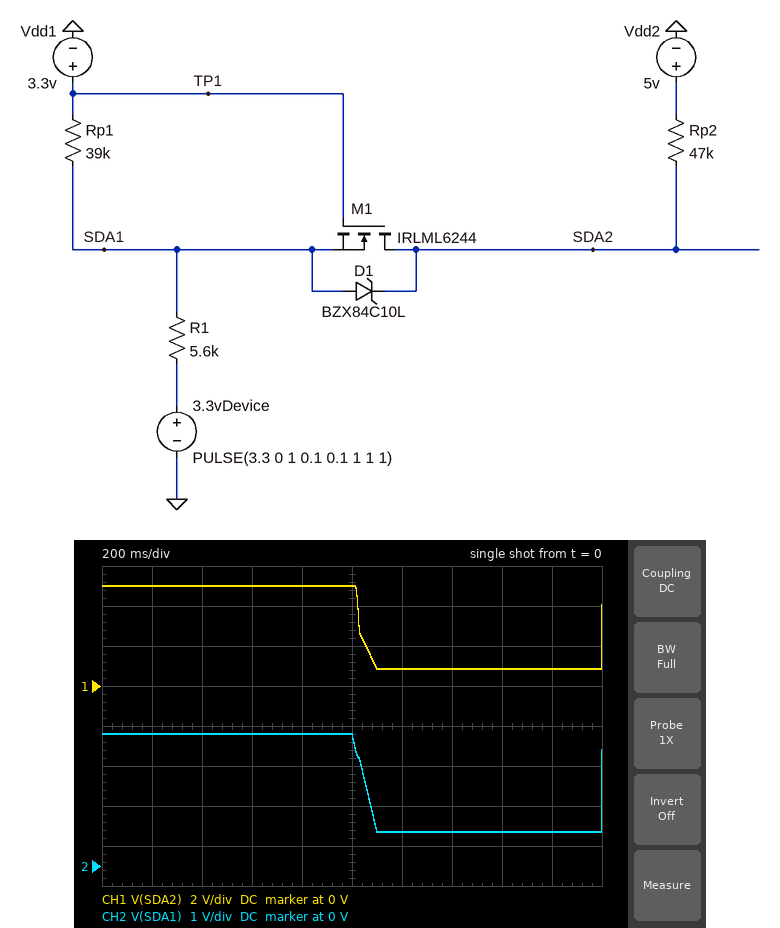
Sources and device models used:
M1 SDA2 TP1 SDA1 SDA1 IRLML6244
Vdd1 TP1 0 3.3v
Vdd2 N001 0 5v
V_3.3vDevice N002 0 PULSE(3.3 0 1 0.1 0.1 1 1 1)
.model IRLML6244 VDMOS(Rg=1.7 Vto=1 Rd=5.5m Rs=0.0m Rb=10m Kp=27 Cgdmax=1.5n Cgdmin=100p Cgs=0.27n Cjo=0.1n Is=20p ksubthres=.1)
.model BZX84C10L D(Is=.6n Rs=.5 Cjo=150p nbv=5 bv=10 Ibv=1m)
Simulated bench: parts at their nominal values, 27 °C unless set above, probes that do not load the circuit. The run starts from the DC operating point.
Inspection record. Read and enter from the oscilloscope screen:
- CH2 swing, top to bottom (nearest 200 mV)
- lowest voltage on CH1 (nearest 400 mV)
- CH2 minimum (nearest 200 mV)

2.4 V
800 mV
800 mV
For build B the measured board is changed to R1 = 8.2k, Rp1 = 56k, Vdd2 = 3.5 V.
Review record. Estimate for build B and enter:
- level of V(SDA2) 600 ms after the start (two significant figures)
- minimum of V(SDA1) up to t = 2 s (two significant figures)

3.5 V
830 mV
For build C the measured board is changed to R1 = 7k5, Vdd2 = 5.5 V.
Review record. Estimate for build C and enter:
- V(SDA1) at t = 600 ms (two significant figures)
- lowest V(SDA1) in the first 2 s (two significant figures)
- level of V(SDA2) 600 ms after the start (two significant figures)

3.3 V
1.1 V
5.5 V
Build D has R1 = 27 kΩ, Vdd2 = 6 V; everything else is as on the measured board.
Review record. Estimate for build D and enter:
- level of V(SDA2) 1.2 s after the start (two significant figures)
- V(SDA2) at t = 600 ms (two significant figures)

2.5 V
6.0 V
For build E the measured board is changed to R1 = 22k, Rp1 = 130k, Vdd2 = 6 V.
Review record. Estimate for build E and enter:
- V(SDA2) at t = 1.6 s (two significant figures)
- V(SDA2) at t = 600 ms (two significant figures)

2.1 V
6.0 V
